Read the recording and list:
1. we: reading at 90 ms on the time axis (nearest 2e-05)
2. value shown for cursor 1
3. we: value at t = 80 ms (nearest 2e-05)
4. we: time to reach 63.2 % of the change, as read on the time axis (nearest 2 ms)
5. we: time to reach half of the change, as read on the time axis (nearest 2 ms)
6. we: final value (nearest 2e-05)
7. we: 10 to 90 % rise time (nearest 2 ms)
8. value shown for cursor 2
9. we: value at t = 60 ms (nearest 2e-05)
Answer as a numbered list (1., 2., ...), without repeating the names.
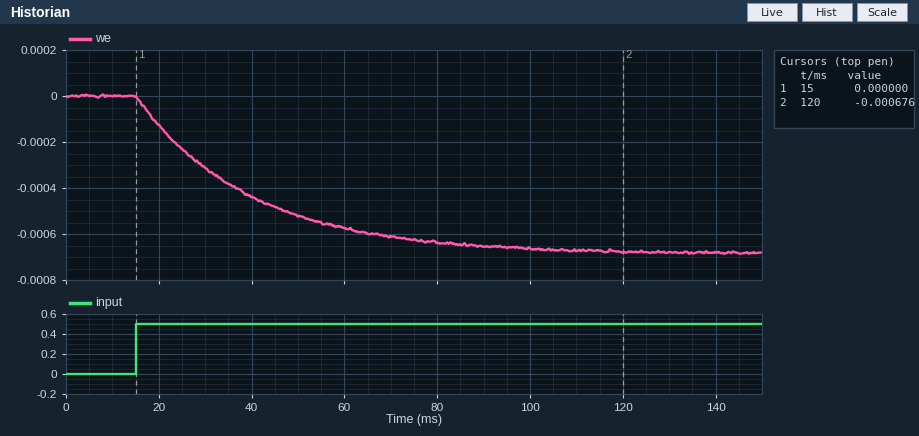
1. -0.00066
2. 0.000000
3. -0.00064
4. 40 ms
5. 32 ms
6. -0.00068
7. 54 ms
8. -0.000676
9. -0.00058
